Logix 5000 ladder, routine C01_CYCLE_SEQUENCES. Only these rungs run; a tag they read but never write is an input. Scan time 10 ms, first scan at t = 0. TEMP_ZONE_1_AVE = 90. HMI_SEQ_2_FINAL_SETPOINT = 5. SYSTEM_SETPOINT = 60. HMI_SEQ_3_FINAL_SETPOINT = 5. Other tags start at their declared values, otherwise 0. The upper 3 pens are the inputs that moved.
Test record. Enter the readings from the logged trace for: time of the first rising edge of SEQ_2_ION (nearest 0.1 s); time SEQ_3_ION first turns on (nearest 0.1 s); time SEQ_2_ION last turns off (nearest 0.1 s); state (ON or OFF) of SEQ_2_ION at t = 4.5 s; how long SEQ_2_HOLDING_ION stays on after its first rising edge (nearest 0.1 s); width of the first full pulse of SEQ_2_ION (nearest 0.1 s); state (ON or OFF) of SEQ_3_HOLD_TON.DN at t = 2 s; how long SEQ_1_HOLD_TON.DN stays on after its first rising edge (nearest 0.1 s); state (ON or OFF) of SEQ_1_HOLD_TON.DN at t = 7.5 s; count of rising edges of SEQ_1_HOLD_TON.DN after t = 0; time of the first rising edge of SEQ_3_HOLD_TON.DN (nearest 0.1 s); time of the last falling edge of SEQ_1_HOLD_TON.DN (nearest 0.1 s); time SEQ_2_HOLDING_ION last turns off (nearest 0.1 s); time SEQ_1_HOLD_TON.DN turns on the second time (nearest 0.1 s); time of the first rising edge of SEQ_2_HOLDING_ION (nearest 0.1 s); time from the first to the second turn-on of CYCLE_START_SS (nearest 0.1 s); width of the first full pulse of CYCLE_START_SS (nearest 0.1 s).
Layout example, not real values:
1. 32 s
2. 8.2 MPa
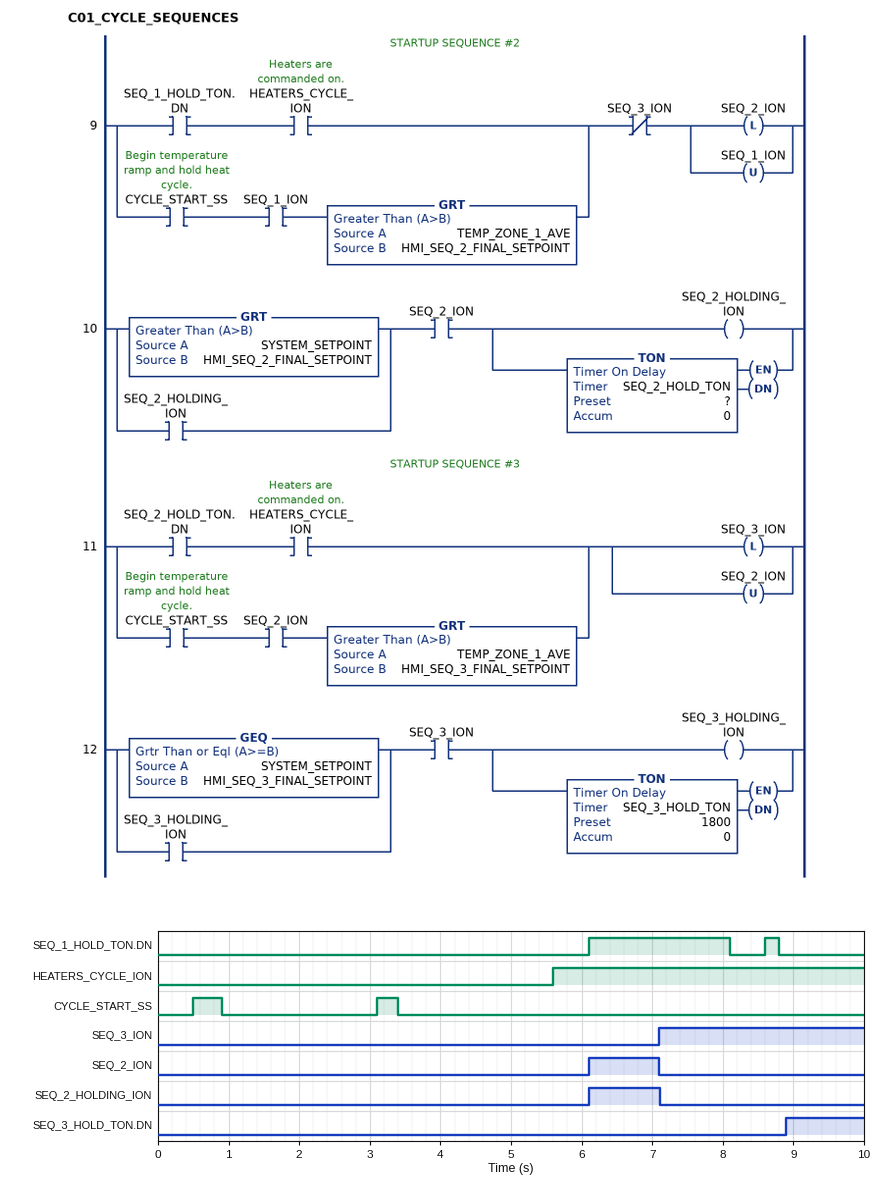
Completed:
1. 6.1 s
2. 7.1 s
3. 7.1 s
4. OFF
5. 1.0 s
6. 1.0 s
7. OFF
8. 2.0 s
9. ON
10. 2
11. 8.9 s
12. 8.8 s
13. 7.1 s
14. 8.6 s
15. 6.1 s
16. 2.6 s
17. 0.4 s
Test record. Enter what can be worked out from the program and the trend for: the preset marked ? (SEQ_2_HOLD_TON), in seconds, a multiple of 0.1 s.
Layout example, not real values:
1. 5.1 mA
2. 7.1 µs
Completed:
1. 1.0 s
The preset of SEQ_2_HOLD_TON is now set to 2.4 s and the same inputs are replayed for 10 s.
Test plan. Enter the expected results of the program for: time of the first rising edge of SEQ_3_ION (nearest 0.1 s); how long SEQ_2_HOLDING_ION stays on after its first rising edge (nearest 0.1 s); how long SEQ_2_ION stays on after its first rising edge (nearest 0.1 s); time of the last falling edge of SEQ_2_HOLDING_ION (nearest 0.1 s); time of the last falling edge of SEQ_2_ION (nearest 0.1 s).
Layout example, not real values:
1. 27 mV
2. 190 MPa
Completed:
1. 8.5 s
2. 2.4 s
3. 2.4 s
4. 8.5 s
5. 8.5 s
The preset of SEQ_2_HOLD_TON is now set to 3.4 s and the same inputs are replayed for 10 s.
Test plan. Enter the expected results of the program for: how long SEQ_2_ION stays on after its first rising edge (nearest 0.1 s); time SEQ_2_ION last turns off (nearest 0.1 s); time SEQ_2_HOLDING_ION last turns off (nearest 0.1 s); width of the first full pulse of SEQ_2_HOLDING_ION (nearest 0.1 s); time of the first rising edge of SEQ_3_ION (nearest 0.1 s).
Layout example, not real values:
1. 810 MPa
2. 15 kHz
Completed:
1. 3.4 s
2. 9.5 s
3. 9.5 s
4. 3.4 s
5. 9.5 s
